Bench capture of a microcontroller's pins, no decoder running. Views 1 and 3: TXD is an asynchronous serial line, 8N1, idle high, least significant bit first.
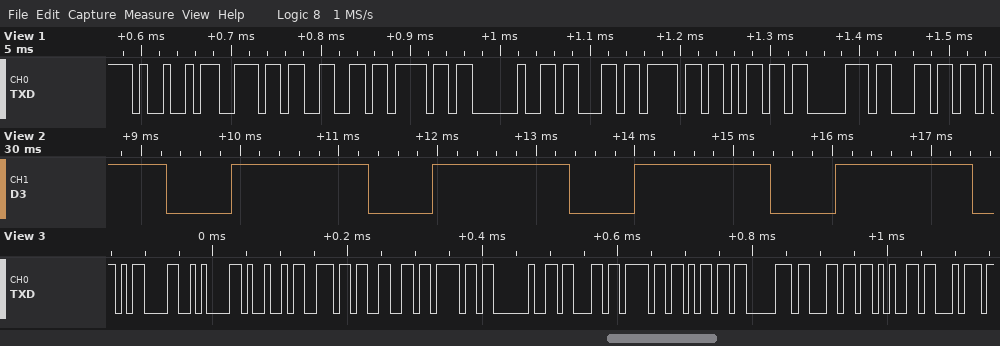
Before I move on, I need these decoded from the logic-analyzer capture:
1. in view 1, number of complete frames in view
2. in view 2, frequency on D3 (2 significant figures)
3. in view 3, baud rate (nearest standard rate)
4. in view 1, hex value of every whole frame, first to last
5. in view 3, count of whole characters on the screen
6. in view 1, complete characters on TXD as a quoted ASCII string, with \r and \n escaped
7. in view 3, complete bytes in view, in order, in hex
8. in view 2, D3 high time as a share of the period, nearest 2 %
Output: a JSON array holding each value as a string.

["10", "490 Hz", "115200 baud", "49 6E 66 6F 20 63 6F 6D 70 6C", "14", "\"Info compl\"", "0D 0A 49 6E 66 6F 20 63 6F 6D 70 6C 65 74", "68 %"]
